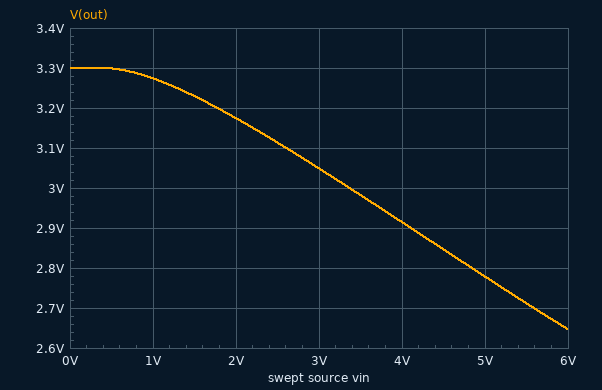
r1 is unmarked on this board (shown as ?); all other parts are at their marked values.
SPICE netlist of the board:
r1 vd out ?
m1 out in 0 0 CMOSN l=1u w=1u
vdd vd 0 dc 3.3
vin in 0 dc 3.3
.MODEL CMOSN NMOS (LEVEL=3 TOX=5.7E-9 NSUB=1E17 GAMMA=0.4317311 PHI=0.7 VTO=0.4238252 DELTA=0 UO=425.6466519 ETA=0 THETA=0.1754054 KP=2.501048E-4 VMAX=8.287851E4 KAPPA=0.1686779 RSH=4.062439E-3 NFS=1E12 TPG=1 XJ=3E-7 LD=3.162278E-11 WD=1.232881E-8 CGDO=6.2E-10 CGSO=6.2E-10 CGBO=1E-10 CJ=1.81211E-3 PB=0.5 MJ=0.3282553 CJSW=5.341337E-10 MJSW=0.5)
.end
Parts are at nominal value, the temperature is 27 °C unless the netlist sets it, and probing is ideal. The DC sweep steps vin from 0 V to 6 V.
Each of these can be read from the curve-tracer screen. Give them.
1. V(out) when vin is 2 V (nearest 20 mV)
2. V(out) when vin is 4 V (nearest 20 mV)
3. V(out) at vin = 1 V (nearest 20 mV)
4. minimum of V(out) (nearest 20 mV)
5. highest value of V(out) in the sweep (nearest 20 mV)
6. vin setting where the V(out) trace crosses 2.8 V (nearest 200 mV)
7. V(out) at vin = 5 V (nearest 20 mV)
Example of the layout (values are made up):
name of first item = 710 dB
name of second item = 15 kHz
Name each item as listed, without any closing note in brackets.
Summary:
V(out) when vin is 2 V = 3.18 V
V(out) when vin is 4 V = 2.92 V
V(out) at vin = 1 V = 3.28 V
minimum of V(out) = 2.64 V
highest value of V(out) in the sweep = 3.30 V
vin setting where the V(out) trace crosses 2.8 V = 4.8 V
V(out) at vin = 5 V = 2.78 V
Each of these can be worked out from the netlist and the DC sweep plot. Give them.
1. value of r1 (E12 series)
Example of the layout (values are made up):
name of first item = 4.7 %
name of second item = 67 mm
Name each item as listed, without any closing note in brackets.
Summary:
value of r1 = 820 Ω
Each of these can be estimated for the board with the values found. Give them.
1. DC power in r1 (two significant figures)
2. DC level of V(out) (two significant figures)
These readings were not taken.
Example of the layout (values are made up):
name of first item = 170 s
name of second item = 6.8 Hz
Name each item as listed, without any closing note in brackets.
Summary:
DC power in r1 = 100 µW
DC level of V(out) = 3.0 V
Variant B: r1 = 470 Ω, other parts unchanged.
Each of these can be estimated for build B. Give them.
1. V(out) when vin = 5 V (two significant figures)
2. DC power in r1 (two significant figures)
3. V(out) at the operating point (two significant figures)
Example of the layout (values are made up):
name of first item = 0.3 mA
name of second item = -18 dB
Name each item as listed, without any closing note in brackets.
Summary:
V(out) when vin = 5 V = 3.0 V
DC power in r1 = 59 µW
V(out) at the operating point = 3.1 V
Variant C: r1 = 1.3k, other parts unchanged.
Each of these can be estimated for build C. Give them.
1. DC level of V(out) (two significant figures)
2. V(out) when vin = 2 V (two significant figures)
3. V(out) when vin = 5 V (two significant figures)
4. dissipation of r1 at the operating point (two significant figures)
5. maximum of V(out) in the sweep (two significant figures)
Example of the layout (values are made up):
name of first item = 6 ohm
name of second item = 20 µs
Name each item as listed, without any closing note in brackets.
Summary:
DC level of V(out) = 2.8 V
V(out) when vin = 2 V = 3.1 V
V(out) when vin = 5 V = 2.5 V
dissipation of r1 at the operating point = 160 µW
maximum of V(out) in the sweep = 3.3 V
